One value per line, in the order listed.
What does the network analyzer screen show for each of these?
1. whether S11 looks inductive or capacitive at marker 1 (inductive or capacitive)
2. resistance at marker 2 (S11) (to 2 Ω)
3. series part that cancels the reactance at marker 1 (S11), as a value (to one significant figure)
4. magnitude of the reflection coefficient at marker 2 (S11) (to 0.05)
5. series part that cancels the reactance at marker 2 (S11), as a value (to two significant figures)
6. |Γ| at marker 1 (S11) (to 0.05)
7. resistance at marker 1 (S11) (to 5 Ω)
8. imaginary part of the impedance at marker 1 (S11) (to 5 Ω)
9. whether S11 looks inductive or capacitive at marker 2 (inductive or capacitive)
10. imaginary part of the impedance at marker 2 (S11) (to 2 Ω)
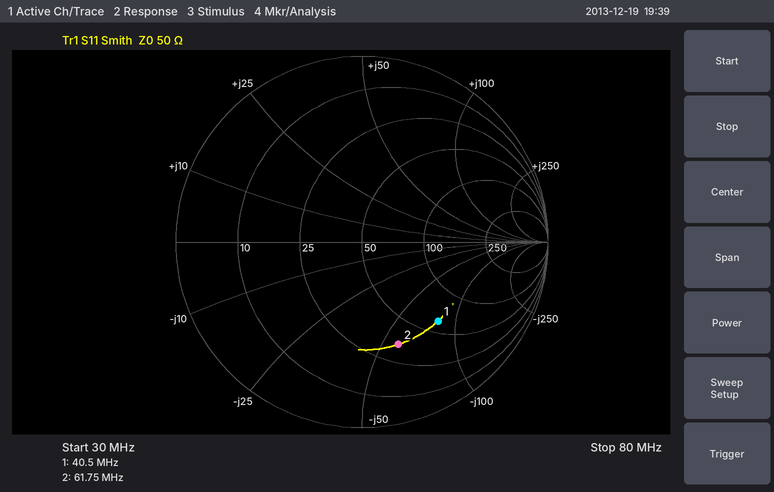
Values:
capacitive
34 Ω
300 nH
0.60
150 nH
0.60
60 Ω
-80 Ω
capacitive
-58 Ω
